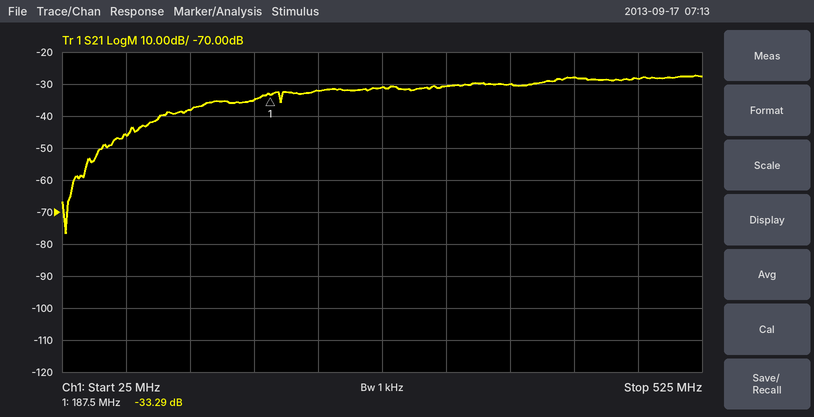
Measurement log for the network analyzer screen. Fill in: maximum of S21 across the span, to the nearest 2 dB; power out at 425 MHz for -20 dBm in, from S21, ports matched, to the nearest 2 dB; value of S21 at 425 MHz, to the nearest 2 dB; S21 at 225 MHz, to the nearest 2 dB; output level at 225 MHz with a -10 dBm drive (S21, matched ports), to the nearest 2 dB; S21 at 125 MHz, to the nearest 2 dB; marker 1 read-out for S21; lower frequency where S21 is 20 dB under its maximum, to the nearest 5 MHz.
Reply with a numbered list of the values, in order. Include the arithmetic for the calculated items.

1. -28 dB
2. -20 dBm + (-28 dB) = -48 dBm
3. -28 dB
4. -32 dB
5. -10 dBm + (-32 dB) = -42 dBm
6. -38 dB
7. -33.29 dB
8. 65 MHz
